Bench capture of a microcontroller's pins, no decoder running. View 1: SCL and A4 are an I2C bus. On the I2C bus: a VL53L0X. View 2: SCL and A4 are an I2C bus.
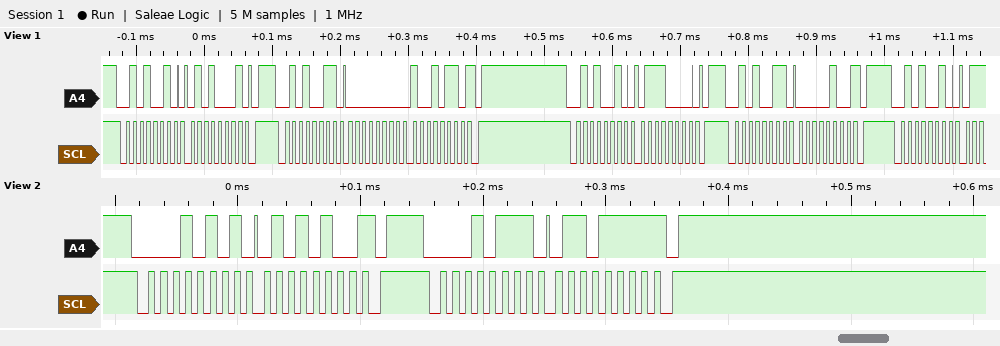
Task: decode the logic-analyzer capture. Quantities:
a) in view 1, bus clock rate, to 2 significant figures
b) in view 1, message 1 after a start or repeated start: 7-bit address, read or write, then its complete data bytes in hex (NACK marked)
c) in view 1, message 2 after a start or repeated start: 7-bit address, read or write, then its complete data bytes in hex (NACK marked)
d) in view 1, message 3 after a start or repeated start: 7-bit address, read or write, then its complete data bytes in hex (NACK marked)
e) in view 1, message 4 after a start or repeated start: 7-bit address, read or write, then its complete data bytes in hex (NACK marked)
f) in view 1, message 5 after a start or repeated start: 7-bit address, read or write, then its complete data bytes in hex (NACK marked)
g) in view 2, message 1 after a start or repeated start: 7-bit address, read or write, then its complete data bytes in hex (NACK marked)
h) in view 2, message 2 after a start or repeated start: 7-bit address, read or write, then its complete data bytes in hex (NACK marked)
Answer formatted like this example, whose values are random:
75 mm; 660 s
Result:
100 kHz; 0x29 write: 51; 0x29 read: 00 96 NACK; 0x29 write: 70; 0x29 read: 04 NACK; 0x29 write; 0x0A read: 54 NACK; 0x0B read: 6F NACK
